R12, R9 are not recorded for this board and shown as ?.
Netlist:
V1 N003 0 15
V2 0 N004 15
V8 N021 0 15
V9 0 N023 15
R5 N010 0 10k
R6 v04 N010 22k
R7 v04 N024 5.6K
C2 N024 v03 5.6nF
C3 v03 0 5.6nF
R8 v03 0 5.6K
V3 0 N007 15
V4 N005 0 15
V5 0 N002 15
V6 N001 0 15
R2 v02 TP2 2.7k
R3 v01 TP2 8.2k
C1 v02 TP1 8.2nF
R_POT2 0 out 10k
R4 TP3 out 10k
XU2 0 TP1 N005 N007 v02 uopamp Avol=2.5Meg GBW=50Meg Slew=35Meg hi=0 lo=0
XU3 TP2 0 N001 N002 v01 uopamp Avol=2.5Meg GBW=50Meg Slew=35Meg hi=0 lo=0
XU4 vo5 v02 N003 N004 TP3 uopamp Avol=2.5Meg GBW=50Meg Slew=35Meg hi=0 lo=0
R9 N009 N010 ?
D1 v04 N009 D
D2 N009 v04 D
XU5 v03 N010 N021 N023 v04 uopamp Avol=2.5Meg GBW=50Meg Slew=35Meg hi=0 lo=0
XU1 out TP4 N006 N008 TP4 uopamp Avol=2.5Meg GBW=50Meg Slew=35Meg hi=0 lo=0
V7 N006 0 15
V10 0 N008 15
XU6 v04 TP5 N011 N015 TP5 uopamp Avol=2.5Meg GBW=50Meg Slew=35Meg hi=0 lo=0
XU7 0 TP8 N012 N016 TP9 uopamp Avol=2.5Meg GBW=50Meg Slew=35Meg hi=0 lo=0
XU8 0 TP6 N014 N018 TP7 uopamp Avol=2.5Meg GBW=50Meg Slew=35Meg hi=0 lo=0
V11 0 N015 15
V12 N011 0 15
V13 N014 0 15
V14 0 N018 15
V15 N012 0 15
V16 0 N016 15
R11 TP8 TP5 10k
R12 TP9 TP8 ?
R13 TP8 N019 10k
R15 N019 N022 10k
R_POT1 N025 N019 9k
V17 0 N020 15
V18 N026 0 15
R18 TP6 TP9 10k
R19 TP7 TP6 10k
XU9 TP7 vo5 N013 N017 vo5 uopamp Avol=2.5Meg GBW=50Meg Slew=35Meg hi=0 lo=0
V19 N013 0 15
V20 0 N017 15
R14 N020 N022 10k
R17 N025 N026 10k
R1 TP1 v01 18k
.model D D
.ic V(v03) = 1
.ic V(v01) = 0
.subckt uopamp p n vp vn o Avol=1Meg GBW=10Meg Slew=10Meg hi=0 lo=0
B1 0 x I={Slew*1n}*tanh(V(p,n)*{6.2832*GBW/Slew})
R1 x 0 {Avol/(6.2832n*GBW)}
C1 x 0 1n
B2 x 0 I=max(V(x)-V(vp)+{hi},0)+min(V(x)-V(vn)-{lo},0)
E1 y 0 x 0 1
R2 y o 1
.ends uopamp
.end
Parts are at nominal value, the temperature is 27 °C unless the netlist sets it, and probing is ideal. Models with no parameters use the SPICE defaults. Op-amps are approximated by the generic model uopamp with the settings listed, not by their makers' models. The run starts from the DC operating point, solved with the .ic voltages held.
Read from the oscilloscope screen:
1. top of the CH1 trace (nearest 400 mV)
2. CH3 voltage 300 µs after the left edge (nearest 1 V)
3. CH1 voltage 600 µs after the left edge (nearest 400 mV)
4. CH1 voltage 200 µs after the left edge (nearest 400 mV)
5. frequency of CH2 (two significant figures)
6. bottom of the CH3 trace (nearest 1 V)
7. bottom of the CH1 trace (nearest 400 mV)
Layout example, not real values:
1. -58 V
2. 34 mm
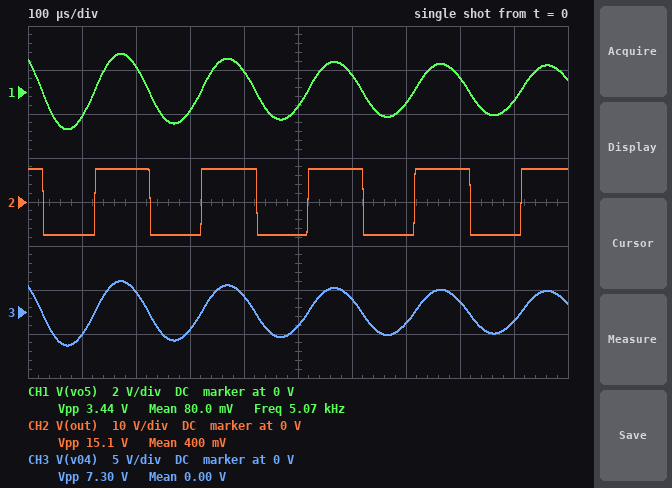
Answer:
1. 1.6 V
2. -2 V
3. 800 mV
4. 1.2 V
5. 5.1 kHz
6. -4 V
7. -1.6 V
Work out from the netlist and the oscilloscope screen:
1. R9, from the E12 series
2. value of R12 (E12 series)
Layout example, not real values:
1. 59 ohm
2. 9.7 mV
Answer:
1. 120 kΩ
2. 4.7 kΩ
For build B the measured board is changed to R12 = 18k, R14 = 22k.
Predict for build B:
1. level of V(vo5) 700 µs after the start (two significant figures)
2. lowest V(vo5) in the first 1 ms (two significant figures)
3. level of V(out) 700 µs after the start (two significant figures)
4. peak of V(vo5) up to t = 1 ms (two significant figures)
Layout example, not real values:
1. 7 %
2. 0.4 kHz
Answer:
1. 810 mV
2. -3.7 V
3. 7.5 V
4. 9.4 V
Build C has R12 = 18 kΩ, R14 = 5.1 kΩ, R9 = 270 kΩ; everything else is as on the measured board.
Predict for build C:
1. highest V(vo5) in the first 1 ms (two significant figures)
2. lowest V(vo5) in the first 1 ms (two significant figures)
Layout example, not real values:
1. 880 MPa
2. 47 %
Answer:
1. 15 V
2. -15 V
